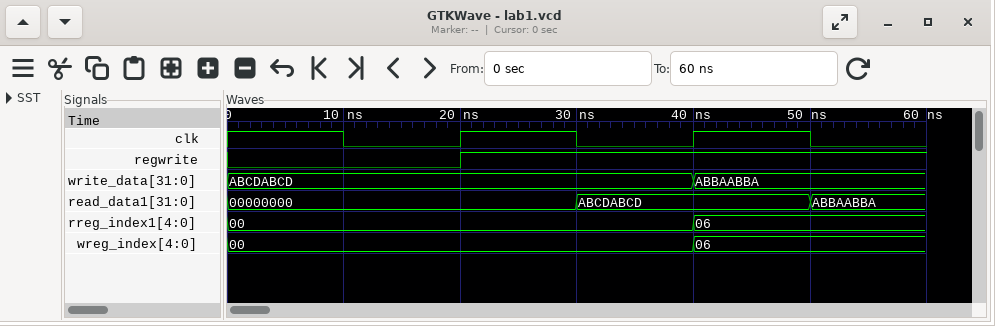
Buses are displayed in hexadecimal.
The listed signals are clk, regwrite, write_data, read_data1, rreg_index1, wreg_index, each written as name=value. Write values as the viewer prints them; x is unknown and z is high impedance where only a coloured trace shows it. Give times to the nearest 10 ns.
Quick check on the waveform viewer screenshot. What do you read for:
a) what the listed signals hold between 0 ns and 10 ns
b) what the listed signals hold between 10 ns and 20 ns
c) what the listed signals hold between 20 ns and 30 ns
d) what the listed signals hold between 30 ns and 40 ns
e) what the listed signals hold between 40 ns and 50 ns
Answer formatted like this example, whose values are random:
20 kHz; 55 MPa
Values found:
clk=1, regwrite=0, write_data=ABCDABCD, read_data1=00000000, rreg_index1=00, wreg_index=00; clk=0, regwrite=0, write_data=ABCDABCD, read_data1=00000000, rreg_index1=00, wreg_index=00; clk=1, regwrite=1, write_data=ABCDABCD, read_data1=00000000, rreg_index1=00, wreg_index=00; clk=0, regwrite=1, write_data=ABCDABCD, read_data1=ABCDABCD, rreg_index1=00, wreg_index=00; clk=1, regwrite=1, write_data=ABBAABBA, read_data1=ABCDABCD, rreg_index1=06, wreg_index=06
